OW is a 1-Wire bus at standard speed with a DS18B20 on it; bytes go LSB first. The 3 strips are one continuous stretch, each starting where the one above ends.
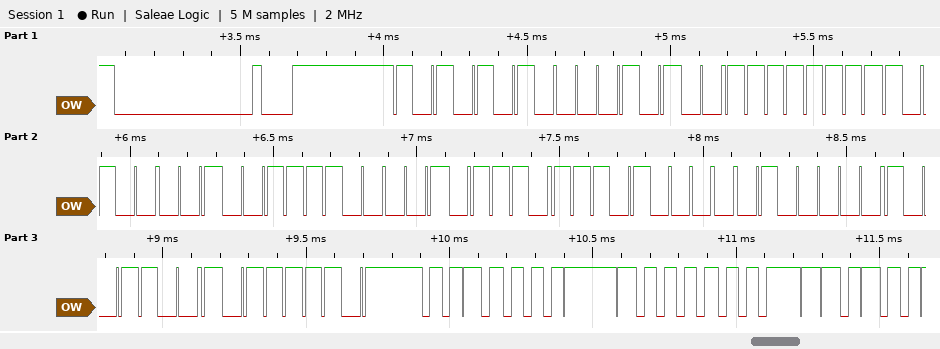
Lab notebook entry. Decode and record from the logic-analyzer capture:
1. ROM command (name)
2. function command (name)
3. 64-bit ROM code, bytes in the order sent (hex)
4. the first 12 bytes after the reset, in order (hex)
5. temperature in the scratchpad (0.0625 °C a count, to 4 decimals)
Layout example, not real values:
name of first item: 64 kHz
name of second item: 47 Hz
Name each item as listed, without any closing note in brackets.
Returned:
ROM command: Match ROM
function command: Read Scratchpad
64-bit ROM code, bytes in the order sent: 28 FF 85 3C 74 17 04 99
the first 12 bytes after the reset, in order: 55 28 FF 85 3C 74 17 04 99 BE 84 01
temperature in the scratchpad: 24.2500 °C
